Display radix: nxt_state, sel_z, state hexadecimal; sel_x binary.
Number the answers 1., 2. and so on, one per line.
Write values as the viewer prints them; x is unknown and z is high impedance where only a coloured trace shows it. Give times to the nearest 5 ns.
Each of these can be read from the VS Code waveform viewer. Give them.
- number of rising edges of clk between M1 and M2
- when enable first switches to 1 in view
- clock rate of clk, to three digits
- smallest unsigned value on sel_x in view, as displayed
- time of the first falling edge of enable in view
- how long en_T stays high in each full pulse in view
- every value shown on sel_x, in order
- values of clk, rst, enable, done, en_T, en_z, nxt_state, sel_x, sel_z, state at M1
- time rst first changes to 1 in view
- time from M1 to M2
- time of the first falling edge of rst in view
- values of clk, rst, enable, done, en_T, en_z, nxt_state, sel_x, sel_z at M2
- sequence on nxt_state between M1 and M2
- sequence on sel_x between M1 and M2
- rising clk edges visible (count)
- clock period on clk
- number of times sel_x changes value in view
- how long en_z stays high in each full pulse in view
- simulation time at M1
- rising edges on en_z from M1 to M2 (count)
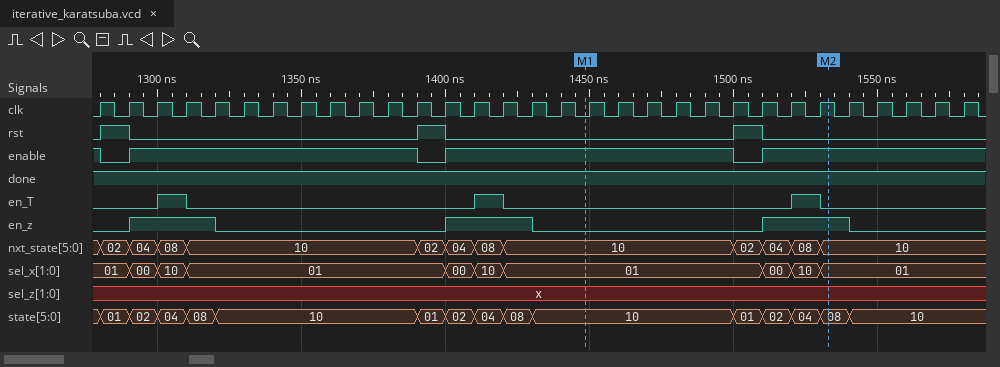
1. 9
2. 1290 ns
3. 100 MHz
4. 00
5. 1280 ns
6. 10 ns, 10 ns, 10 ns
7. 01, 00, 10, 01, 00, 10, 01, 00, 10, 01
8. clk=0, rst=0, enable=1, done=1, en_T=0, en_z=0, nxt_state=10, sel_x=01, sel_z=x, state=10
9. 1280 ns
10. 85 ns
11. 1290 ns
12. clk=1, rst=0, enable=1, done=1, en_T=0, en_z=1, nxt_state=10, sel_x=01, sel_z=x
13. 10, 02, 04, 08, 10
14. 01, 00, 10, 01
15. 31
16. 10 ns
17. 9
18. 30 ns, 30 ns, 30 ns
19. 1450 ns
20. 1
